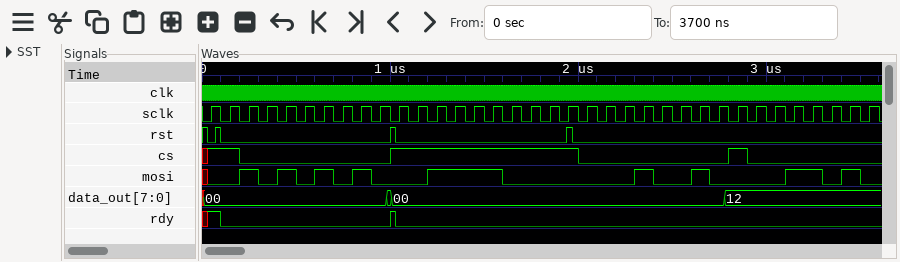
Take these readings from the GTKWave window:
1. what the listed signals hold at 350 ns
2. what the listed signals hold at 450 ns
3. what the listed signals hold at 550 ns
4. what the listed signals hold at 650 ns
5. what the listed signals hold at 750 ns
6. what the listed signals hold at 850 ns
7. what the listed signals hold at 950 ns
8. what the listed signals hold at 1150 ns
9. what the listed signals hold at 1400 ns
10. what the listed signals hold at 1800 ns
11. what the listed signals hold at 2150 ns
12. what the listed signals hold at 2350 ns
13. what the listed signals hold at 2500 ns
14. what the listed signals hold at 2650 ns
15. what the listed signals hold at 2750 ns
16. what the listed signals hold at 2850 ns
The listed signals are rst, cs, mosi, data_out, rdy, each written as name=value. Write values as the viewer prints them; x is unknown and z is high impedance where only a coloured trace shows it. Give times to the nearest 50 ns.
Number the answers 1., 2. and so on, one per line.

1. rst=0, cs=0, mosi=0, data_out=00, rdy=0
2. rst=0, cs=0, mosi=1, data_out=00, rdy=0
3. rst=0, cs=0, mosi=0, data_out=00, rdy=0
4. rst=0, cs=0, mosi=1, data_out=00, rdy=0
5. rst=0, cs=0, mosi=0, data_out=00, rdy=0
6. rst=0, cs=0, mosi=1, data_out=00, rdy=0
7. rst=0, cs=0, mosi=0, data_out=00, rdy=0
8. rst=0, cs=1, mosi=0, data_out=00, rdy=0
9. rst=0, cs=1, mosi=1, data_out=00, rdy=0
10. rst=0, cs=1, mosi=0, data_out=00, rdy=0
11. rst=0, cs=0, mosi=0, data_out=00, rdy=0
12. rst=0, cs=0, mosi=1, data_out=00, rdy=0
13. rst=0, cs=0, mosi=0, data_out=00, rdy=0
14. rst=0, cs=0, mosi=1, data_out=00, rdy=0
15. rst=0, cs=0, mosi=0, data_out=00, rdy=0
16. rst=0, cs=1, mosi=0, data_out=12, rdy=0
